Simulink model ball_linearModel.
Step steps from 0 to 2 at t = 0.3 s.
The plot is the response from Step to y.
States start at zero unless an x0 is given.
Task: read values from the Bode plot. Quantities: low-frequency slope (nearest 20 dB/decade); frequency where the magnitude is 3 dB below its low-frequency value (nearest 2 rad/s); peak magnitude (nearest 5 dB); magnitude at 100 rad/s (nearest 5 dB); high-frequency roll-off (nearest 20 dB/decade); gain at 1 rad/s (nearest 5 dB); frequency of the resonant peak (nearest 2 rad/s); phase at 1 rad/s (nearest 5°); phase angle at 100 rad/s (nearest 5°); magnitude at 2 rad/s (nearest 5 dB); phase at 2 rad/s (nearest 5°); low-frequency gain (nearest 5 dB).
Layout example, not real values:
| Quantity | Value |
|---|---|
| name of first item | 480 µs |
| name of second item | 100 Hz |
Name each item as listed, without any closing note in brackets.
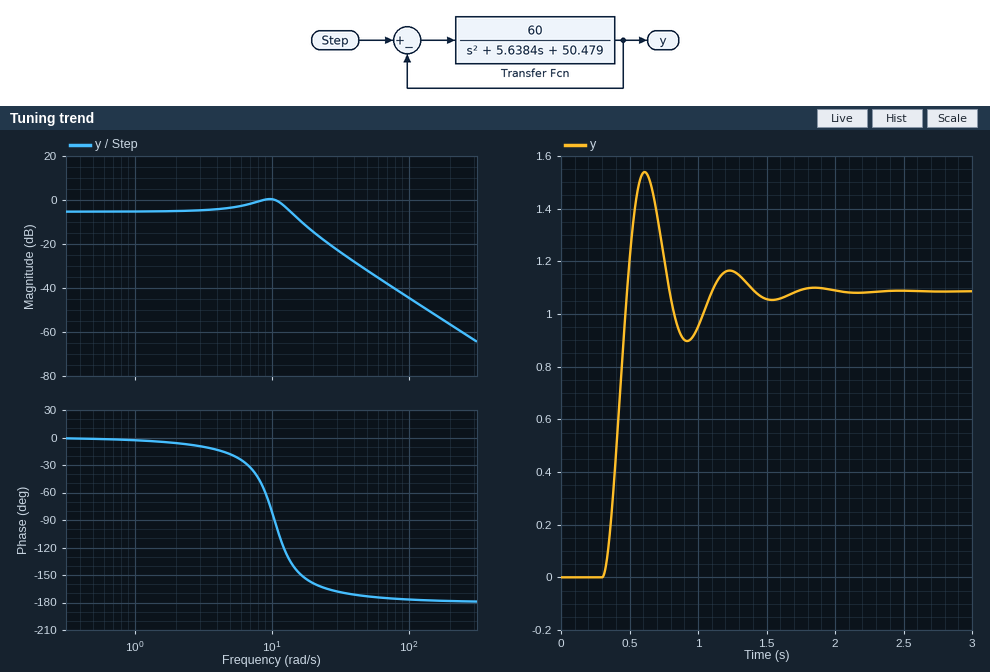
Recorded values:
| Quantity | Value |
|---|---|
| low-frequency slope | 0 dB/decade |
| frequency where the magnitude is 3 dB below its low-frequency value | 16 rad/s |
| peak magnitude | 0 dB |
| magnitude at 100 rad/s | -45 dB |
| high-frequency roll-off | -40 dB/decade |
| gain at 1 rad/s | -5 dB |
| frequency of the resonant peak | 10 rad/s |
| phase at 1 rad/s | -5° |
| phase angle at 100 rad/s | -175° |
| magnitude at 2 rad/s | -5 dB |
| phase at 2 rad/s | -5° |
| low-frequency gain | -5 dB |
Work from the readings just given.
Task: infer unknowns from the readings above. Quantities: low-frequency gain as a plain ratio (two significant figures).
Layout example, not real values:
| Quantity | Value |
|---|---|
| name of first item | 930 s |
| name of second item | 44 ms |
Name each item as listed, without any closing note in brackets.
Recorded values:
| Quantity | Value |
|---|---|
| low-frequency gain as a plain ratio | 0.56 |
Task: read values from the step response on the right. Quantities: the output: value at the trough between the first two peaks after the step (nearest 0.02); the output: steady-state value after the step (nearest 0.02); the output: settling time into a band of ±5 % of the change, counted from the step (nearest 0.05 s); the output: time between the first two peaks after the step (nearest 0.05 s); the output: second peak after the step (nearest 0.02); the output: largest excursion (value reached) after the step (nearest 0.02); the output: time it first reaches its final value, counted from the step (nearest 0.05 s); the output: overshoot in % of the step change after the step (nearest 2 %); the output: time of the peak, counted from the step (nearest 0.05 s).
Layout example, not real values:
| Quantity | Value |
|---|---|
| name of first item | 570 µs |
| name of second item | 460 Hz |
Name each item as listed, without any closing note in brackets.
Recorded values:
| Quantity | Value |
|---|---|
| the output: value at the trough between the first two peaks after the step | 0.90 |
| the output: steady-state value after the step | 1.08 |
| the output: settling time into a band of ±5 % of the change, counted from the step | 1.00 s |
| the output: time between the first two peaks after the step | 0.60 s |
| the output: second peak after the step | 1.16 |
| the output: largest excursion (value reached) after the step | 1.54 |
| the output: time it first reaches its final value, counted from the step | 0.20 s |
| the output: overshoot in % of the step change after the step | 42 % |
| the output: time of the peak, counted from the step | 0.30 s |
